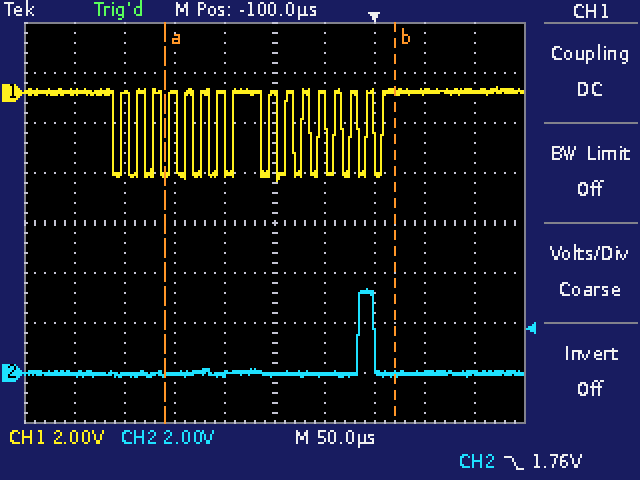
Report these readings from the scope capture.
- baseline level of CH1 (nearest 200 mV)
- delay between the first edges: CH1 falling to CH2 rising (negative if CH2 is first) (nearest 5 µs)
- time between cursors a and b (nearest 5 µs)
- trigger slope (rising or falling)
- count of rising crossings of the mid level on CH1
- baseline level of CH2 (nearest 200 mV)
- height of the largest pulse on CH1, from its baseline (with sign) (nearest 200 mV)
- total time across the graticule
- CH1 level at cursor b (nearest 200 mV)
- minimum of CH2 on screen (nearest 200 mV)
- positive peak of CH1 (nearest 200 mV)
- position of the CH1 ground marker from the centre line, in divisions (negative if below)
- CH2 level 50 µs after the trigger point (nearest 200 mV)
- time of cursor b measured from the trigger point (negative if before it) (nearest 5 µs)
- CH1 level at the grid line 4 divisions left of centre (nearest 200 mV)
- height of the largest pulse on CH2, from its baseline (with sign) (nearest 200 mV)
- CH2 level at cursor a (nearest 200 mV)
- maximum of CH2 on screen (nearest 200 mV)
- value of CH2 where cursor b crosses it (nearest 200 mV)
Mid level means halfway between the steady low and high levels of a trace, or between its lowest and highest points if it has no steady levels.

0.0 V
+245 µs
230 µs
falling
16
0.0 V
-3.6 V
500 µs
0.0 V
-200 mV
200 mV
+2.6 div
0.0 V
+20 µs
0.0 V
+3.4 V
0.0 V
3.4 V
0.0 V
